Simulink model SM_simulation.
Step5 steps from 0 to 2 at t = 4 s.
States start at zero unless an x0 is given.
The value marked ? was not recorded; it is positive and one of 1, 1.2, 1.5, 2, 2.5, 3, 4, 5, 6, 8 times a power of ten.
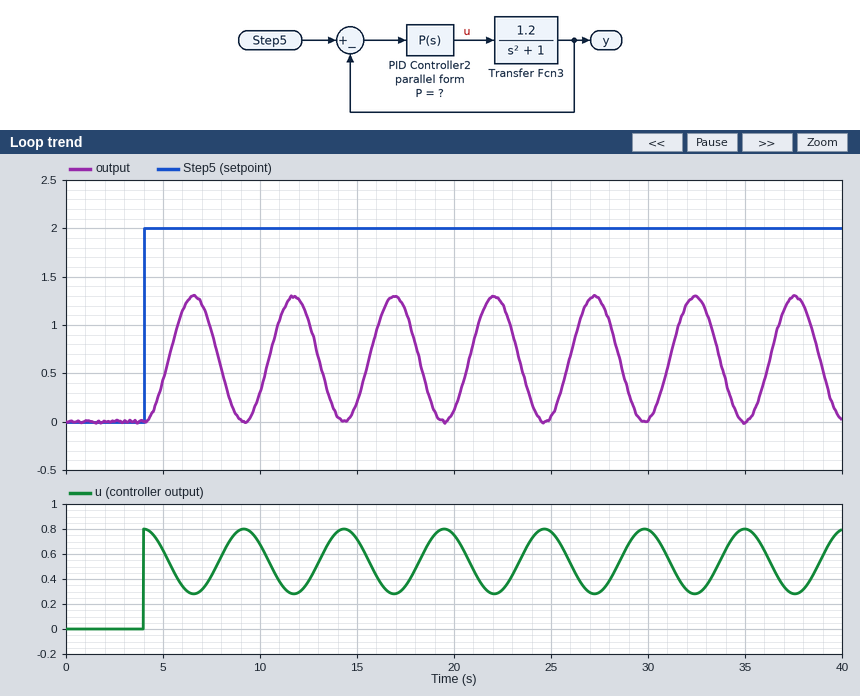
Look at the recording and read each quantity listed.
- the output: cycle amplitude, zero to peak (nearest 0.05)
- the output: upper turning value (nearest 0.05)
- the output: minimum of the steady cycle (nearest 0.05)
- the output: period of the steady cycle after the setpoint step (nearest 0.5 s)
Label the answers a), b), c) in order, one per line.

a) 0.65
b) 1.30
c) 0.00
d) 5.0 s
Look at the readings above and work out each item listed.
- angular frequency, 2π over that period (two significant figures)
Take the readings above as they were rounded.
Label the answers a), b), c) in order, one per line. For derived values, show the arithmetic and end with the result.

a) 2π / 5 = 1.3 rad/s
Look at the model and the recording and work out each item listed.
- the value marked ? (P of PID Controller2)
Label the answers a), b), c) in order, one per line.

a) 0.4
